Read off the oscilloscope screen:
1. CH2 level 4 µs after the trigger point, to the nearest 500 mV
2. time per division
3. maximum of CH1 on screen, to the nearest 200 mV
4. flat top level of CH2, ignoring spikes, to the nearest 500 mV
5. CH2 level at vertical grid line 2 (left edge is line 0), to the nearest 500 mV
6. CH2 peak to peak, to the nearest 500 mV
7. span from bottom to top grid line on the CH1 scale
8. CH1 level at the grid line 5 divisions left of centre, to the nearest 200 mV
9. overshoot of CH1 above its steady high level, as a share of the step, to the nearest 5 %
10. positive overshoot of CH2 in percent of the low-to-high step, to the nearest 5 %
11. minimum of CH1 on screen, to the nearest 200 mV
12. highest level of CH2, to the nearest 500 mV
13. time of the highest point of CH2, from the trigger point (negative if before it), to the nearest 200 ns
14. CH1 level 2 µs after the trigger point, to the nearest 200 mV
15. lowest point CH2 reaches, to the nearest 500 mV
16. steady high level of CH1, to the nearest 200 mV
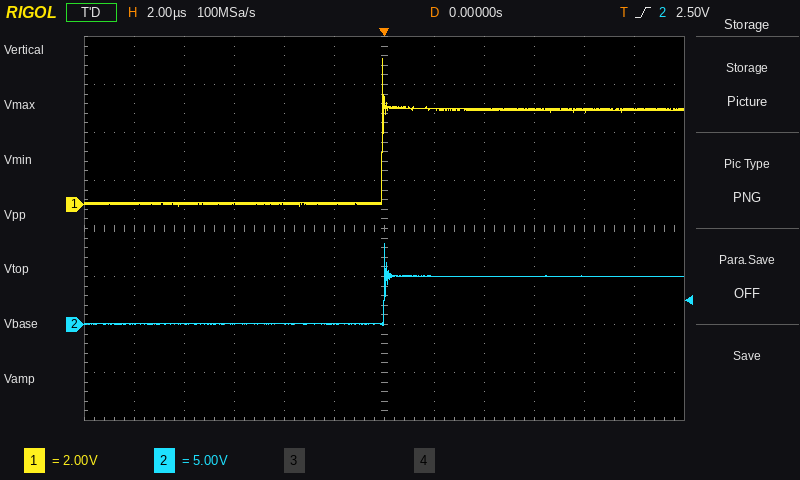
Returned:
5.0 V
2 µs
6.0 V
5.0 V
0.0 V
8.5 V
16 V
0.0 V
55 %
70 %
0.0 V
8.5 V
0.0 µs
4.0 V
0.0 V
4.0 V
